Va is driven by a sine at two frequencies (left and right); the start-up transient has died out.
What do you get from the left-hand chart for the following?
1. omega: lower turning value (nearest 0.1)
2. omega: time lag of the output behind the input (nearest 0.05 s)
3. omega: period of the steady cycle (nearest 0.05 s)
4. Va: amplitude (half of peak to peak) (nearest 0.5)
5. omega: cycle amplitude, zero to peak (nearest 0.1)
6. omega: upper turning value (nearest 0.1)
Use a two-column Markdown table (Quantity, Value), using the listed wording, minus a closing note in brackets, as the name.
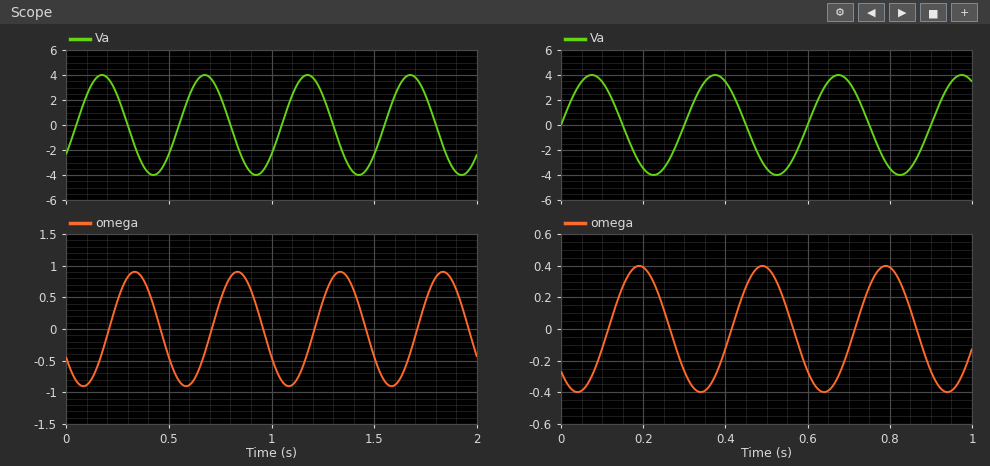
| Quantity | Value |
|---|---|
| omega: lower turning value | -0.9 |
| omega: time lag of the output behind the input | 0.15 s |
| omega: period of the steady cycle | 0.50 s |
| Va: amplitude (half of peak to peak) | 4.0 |
| omega: cycle amplitude, zero to peak | 0.9 |
| omega: upper turning value | 0.9 |
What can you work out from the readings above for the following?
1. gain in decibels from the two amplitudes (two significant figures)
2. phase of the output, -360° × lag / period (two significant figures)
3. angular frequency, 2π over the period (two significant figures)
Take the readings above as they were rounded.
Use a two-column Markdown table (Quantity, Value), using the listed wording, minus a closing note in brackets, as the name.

| Quantity | Value |
|---|---|
| gain in decibels from the two amplitudes | -13 dB |
| phase of the output, -360° × lag / period | -110° |
| angular frequency, 2π over the period | 13 rad/s |
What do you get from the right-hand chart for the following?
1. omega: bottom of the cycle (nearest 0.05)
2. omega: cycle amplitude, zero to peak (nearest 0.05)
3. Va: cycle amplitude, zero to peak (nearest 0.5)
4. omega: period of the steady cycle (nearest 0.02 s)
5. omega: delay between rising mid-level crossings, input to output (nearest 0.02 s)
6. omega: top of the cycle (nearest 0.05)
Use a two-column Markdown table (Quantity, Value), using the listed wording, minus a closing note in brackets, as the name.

| Quantity | Value |
|---|---|
| omega: bottom of the cycle | -0.40 |
| omega: cycle amplitude, zero to peak | 0.40 |
| Va: cycle amplitude, zero to peak | 4.0 |
| omega: period of the steady cycle | 0.30 s |
| omega: delay between rising mid-level crossings, input to output | 0.12 s |
| omega: top of the cycle | 0.40 |
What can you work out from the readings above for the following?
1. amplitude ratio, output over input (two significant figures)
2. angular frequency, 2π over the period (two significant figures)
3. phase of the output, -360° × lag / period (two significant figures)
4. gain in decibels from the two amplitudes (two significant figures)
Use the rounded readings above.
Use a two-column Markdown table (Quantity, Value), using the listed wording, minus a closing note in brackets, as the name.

| Quantity | Value |
|---|---|
| amplitude ratio, output over input | 0.10 |
| angular frequency, 2π over the period | 21 rad/s |
| phase of the output, -360° × lag / period | -140° |
| gain in decibels from the two amplitudes | -20 dB |
